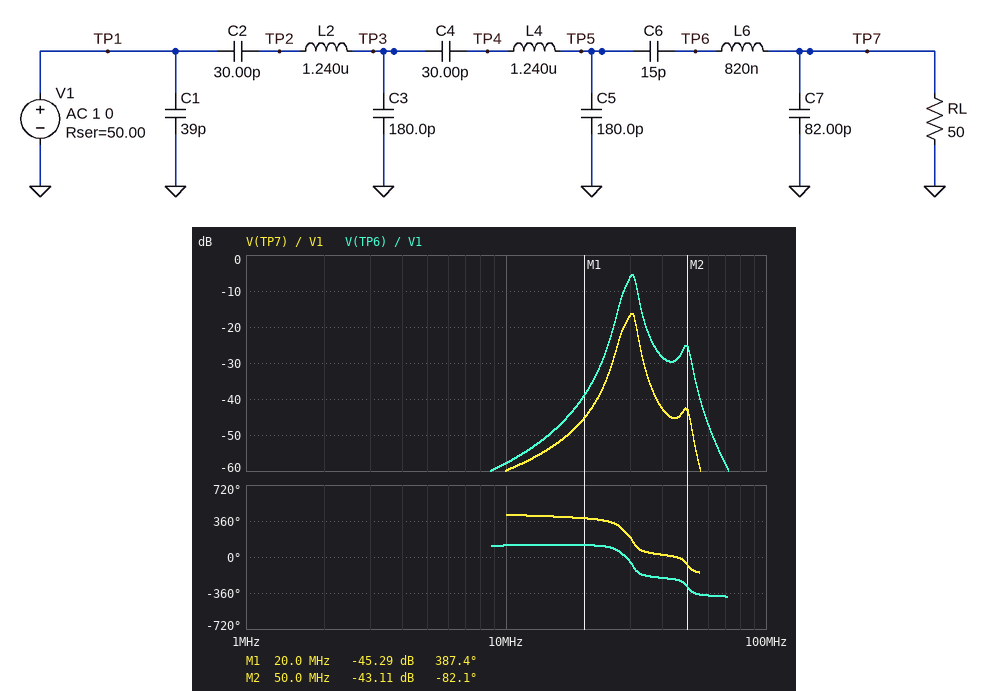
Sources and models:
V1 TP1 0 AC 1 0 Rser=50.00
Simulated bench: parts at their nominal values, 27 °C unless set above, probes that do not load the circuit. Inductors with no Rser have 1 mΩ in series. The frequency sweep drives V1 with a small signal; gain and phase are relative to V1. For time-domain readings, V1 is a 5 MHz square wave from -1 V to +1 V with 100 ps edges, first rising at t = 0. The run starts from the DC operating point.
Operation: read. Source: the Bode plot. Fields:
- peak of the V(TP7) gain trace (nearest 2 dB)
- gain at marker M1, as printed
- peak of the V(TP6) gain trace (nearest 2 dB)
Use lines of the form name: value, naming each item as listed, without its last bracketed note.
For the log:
peak of the V(TP7) gain trace: -16 dB
gain at marker M1, as printed: -45.29 dB
peak of the V(TP6) gain trace: -6 dB
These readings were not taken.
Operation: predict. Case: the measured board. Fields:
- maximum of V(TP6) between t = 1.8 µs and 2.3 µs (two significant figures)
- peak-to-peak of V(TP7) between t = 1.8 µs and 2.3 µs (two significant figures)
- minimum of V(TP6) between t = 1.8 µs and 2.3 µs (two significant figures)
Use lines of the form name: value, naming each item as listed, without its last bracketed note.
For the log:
maximum of V(TP6) between t = 1.8 µs and 2.3 µs: 33 mV
peak-to-peak of V(TP7) between t = 1.8 µs and 2.3 µs: 20 mV
minimum of V(TP6) between t = 1.8 µs and 2.3 µs: -33 mV
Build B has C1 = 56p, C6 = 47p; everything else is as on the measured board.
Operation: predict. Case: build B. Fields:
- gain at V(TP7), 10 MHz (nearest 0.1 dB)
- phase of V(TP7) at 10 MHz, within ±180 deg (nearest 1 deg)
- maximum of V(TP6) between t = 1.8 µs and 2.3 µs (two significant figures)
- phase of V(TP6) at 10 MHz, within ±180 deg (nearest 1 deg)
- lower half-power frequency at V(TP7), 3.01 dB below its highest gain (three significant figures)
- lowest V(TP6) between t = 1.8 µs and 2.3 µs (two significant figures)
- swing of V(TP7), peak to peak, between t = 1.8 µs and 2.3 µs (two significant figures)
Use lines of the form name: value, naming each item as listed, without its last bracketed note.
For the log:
gain at V(TP7), 10 MHz: -50.7 dB
phase of V(TP7) at 10 MHz, within ±180 deg: 53 deg
maximum of V(TP6) between t = 1.8 µs and 2.3 µs: 170 mV
phase of V(TP6) at 10 MHz, within ±180 deg: 108 deg
lower half-power frequency at V(TP7), 3.01 dB below its highest gain: 26.9 MHz
lowest V(TP6) between t = 1.8 µs and 2.3 µs: -170 mV
swing of V(TP7), peak to peak, between t = 1.8 µs and 2.3 µs: 110 mV
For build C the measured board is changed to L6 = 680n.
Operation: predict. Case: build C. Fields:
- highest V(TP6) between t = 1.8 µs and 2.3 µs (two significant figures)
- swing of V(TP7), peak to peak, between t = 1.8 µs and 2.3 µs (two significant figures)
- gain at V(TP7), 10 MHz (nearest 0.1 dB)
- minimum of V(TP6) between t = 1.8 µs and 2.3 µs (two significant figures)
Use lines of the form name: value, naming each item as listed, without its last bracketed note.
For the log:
highest V(TP6) between t = 1.8 µs and 2.3 µs: 23 mV
swing of V(TP7), peak to peak, between t = 1.8 µs and 2.3 µs: 18 mV
gain at V(TP7), 10 MHz: -60.0 dB
minimum of V(TP6) between t = 1.8 µs and 2.3 µs: -23 mV
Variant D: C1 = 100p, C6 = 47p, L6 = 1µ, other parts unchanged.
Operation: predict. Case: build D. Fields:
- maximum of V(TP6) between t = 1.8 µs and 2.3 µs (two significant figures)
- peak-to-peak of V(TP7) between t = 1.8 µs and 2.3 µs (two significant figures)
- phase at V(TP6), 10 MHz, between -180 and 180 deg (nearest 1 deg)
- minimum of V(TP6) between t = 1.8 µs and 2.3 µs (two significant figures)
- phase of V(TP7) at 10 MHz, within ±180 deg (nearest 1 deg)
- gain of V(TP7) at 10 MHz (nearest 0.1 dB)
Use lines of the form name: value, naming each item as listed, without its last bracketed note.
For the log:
maximum of V(TP6) between t = 1.8 µs and 2.3 µs: 190 mV
peak-to-peak of V(TP7) between t = 1.8 µs and 2.3 µs: 110 mV
phase at V(TP6), 10 MHz, between -180 and 180 deg: 108 deg
minimum of V(TP6) between t = 1.8 µs and 2.3 µs: -190 mV
phase of V(TP7) at 10 MHz, within ±180 deg: 46 deg
gain of V(TP7) at 10 MHz: -50.8 dB
